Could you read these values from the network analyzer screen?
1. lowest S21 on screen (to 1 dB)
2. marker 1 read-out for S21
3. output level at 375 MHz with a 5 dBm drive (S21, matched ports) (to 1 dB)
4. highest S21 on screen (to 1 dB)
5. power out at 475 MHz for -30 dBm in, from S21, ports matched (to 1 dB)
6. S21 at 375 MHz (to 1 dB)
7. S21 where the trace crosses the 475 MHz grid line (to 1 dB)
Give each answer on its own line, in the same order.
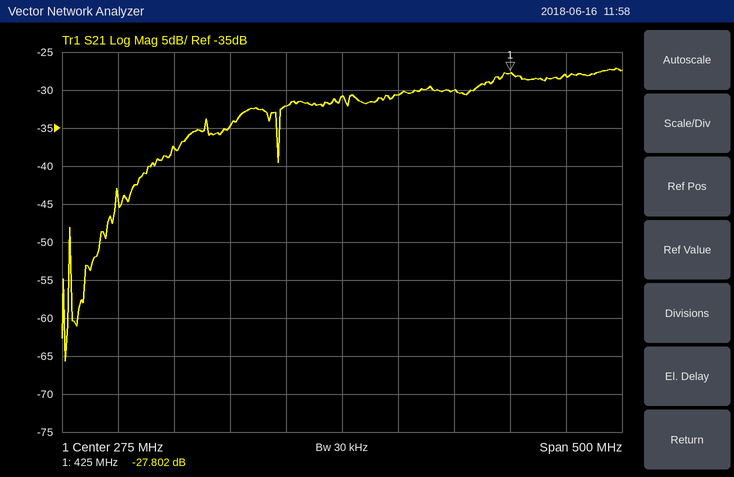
-66 dB
-27.802 dB
-25 dBm
-27 dB
-58 dBm
-30 dB
-28 dB
